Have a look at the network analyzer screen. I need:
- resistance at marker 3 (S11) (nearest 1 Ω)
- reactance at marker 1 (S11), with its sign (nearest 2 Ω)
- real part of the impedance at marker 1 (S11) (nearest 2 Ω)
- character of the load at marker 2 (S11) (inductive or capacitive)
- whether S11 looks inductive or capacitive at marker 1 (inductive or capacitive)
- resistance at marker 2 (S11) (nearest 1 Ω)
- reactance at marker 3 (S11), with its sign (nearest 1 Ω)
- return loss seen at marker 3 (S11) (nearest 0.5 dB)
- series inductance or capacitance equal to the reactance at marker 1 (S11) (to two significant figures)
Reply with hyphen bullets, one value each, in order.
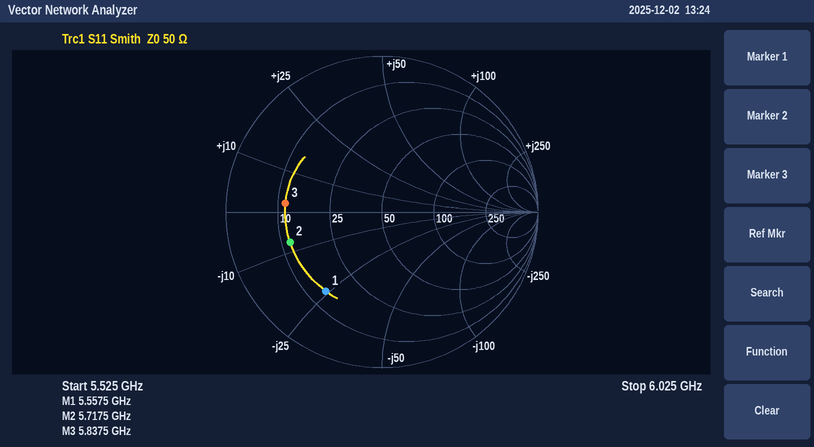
- 12 Ω
- -24 Ω
- 14 Ω
- capacitive
- capacitive
- 12 Ω
- +2 Ω
- 4.0 dB
- 1.2 pF
